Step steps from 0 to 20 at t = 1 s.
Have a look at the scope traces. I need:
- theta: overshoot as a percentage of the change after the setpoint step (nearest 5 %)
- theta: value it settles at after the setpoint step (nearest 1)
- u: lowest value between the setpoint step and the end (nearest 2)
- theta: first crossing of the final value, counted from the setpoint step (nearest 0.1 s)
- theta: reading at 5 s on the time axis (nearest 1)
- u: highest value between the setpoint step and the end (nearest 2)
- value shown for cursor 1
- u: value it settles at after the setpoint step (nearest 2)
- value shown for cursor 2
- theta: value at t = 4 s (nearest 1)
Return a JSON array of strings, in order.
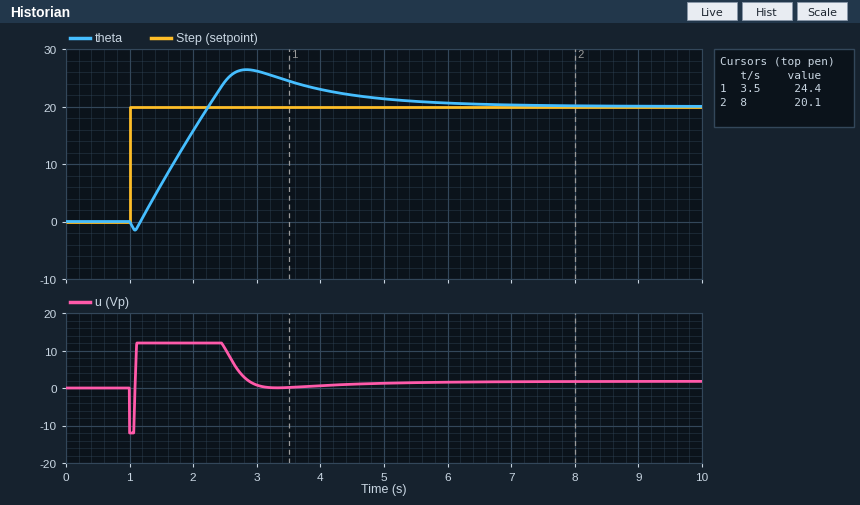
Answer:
["30 %", "20", "-12", "1.2 s", "21", "12", "24.4", "2", "20.1", "23"]
